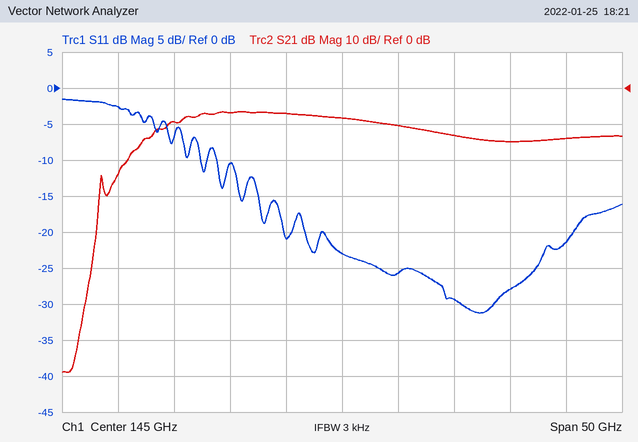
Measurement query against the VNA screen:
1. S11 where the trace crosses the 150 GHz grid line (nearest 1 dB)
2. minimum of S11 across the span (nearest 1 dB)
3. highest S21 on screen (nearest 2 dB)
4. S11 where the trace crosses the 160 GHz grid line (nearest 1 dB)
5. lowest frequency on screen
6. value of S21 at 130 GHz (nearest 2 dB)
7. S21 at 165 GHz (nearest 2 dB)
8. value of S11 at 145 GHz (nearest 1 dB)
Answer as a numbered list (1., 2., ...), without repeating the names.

1. -26 dB
2. -31 dB
3. -6 dB
4. -28 dB
5. 120 GHz
6. -10 dB
7. -14 dB
8. -23 dB
